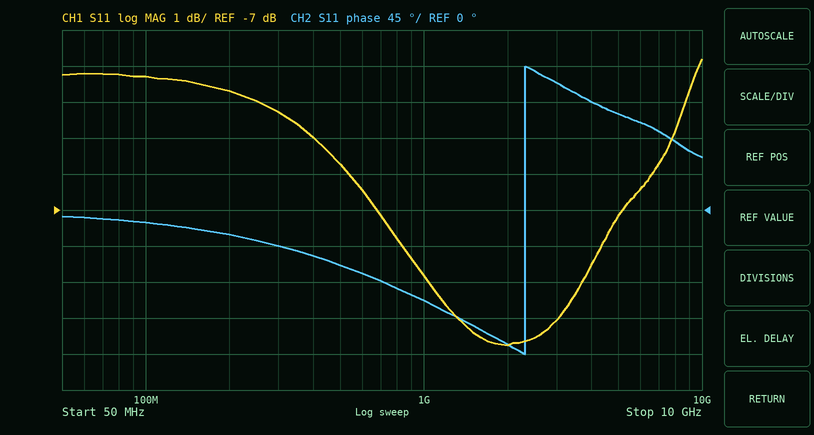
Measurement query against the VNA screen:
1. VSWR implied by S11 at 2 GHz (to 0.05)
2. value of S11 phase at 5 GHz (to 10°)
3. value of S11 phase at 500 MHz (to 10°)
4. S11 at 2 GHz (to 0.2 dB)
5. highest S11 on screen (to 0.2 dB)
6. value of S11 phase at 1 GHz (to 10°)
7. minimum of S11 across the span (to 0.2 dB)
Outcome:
1.80
120°
-70°
-10.8 dB
-2.8 dB
-110°
-10.8 dB
